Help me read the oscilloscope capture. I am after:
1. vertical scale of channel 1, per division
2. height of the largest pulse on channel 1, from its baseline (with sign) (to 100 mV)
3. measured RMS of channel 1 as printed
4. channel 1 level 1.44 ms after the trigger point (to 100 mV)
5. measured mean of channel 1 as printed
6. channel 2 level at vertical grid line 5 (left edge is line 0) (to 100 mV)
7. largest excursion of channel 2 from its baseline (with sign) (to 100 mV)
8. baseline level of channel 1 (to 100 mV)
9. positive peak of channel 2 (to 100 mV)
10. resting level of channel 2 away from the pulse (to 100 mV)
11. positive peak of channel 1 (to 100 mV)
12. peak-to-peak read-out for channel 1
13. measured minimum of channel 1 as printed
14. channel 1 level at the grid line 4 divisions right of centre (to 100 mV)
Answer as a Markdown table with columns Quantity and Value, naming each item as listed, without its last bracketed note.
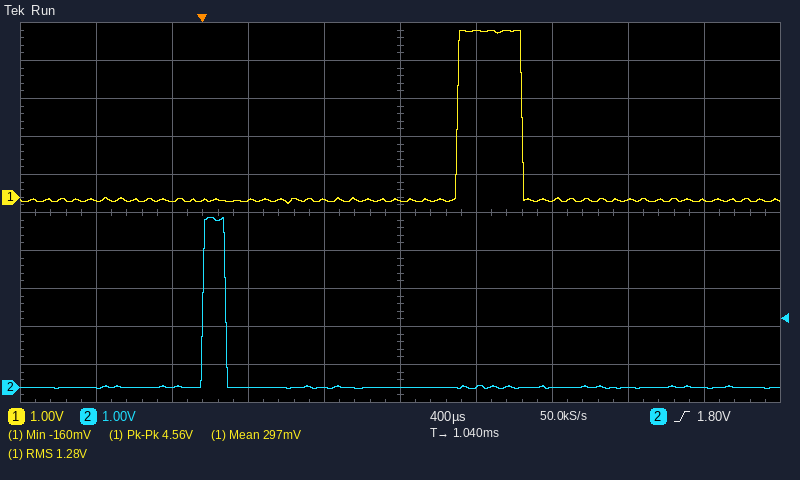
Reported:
| Quantity | Value |
|---|---|
| vertical scale of channel 1, per division | 1 V |
| height of the largest pulse on channel 1, from its baseline (with sign) | +4.5 V |
| measured RMS of channel 1 as printed | 1.28 V |
| channel 1 level 1.44 ms after the trigger point | 4.4 V |
| measured mean of channel 1 as printed | 297 mV |
| channel 2 level at vertical grid line 5 (left edge is line 0) | 0.0 V |
| largest excursion of channel 2 from its baseline (with sign) | +4.5 V |
| baseline level of channel 1 | -100 mV |
| positive peak of channel 2 | 4.5 V |
| resting level of channel 2 away from the pulse | 0.0 V |
| positive peak of channel 1 | 4.4 V |
| peak-to-peak read-out for channel 1 | 4.56 V |
| measured minimum of channel 1 as printed | -160 mV |
| channel 1 level at the grid line 4 divisions right of centre | -100 mV |
